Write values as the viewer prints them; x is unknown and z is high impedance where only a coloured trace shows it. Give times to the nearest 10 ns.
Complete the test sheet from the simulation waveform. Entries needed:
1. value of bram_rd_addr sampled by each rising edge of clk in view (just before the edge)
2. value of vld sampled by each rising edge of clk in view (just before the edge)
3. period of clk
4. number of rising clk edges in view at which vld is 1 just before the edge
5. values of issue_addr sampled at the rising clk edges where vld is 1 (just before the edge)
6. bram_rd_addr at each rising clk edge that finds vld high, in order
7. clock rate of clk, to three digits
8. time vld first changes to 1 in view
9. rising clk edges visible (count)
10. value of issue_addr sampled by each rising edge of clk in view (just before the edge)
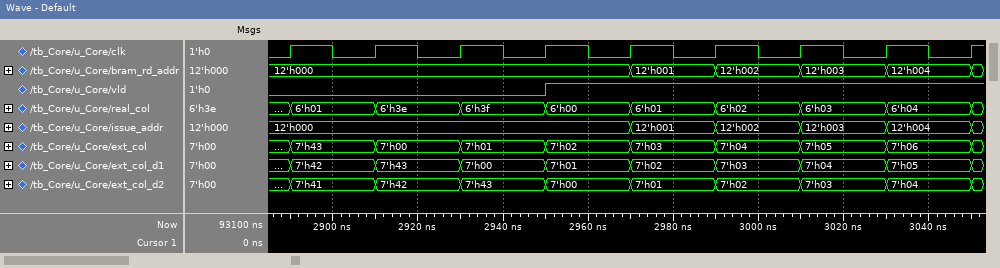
12'h000, 12'h000, 12'h000, 12'h000, 12'h000, 12'h001, 12'h002, 12'h003, 12'h004
0 0 0 0 1 1 1 1 1
20 ns
5
12'h000, 12'h001, 12'h002, 12'h003, 12'h004
12'h000, 12'h001, 12'h002, 12'h003, 12'h004
50.0 MHz
2950 ns
9
12'h000, 12'h000, 12'h000, 12'h000, 12'h000, 12'h001, 12'h002, 12'h003, 12'h004
